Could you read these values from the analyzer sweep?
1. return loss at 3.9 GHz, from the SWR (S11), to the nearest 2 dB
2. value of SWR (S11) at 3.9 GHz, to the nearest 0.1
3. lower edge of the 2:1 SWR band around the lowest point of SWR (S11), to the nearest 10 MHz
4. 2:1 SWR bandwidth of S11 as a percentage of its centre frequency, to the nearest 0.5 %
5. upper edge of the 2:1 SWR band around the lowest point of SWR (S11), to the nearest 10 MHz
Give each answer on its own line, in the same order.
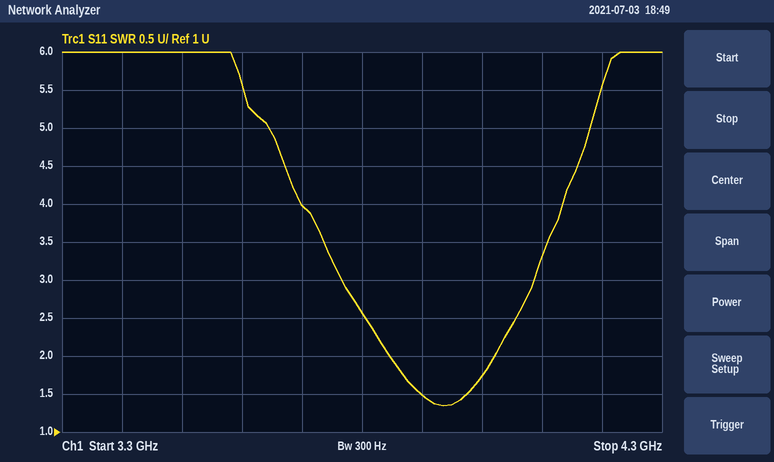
14 dB
1.5
3.85 GHz
4.5 %
4.02 GHz
